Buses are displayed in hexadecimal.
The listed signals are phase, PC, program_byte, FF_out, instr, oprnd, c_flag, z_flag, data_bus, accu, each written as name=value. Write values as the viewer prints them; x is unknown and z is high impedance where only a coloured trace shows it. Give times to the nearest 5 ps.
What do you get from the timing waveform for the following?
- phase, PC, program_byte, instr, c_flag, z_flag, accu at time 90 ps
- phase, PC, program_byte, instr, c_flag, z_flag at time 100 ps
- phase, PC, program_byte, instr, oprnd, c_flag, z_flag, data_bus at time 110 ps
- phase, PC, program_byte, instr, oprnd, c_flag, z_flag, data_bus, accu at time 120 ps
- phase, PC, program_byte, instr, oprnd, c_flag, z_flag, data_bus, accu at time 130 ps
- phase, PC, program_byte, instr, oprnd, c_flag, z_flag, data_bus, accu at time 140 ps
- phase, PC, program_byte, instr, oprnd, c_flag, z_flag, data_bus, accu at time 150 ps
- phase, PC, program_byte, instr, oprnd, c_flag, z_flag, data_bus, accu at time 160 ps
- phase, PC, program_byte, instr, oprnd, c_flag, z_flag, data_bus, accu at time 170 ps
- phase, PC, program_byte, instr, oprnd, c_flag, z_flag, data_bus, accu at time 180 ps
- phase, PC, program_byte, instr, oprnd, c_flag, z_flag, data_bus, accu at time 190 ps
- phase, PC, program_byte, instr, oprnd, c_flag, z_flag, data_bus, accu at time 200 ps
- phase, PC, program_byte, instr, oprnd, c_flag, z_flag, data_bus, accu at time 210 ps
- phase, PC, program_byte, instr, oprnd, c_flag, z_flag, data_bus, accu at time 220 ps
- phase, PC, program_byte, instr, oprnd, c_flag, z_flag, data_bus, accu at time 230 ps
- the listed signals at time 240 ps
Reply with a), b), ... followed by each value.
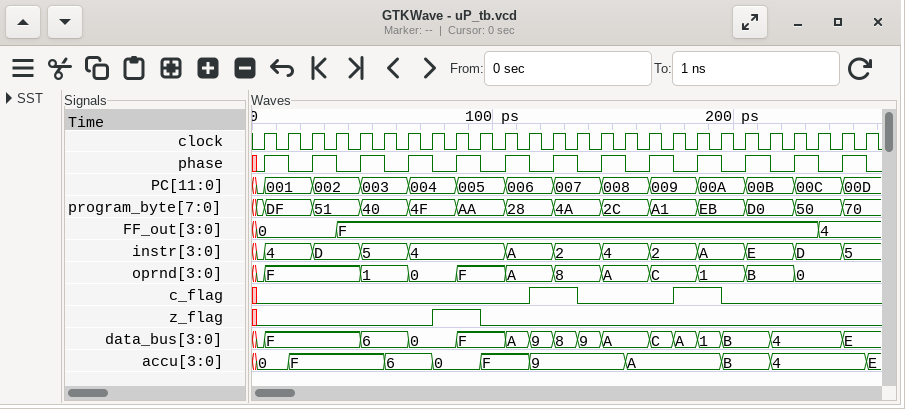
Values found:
a) phase=1, PC=005, program_byte=AA, instr=4, c_flag=0, z_flag=1, accu=0
b) phase=0, PC=005, program_byte=AA, instr=4, c_flag=0, z_flag=0
c) phase=1, PC=006, program_byte=28, instr=A, oprnd=A, c_flag=0, z_flag=0, data_bus=A
d) phase=0, PC=006, program_byte=28, instr=A, oprnd=A, c_flag=1, z_flag=0, data_bus=9, accu=9
e) phase=1, PC=007, program_byte=4A, instr=2, oprnd=8, c_flag=1, z_flag=0, data_bus=8, accu=9
f) phase=0, PC=007, program_byte=4A, instr=2, oprnd=8, c_flag=0, z_flag=0, data_bus=9, accu=9
g) phase=1, PC=008, program_byte=2C, instr=4, oprnd=A, c_flag=0, z_flag=0, data_bus=A, accu=9
h) phase=0, PC=008, program_byte=2C, instr=4, oprnd=A, c_flag=0, z_flag=0, data_bus=A, accu=A
i) phase=1, PC=009, program_byte=A1, instr=2, oprnd=C, c_flag=0, z_flag=0, data_bus=C, accu=A
j) phase=0, PC=009, program_byte=A1, instr=2, oprnd=C, c_flag=1, z_flag=0, data_bus=A, accu=A
k) phase=1, PC=00A, program_byte=EB, instr=A, oprnd=1, c_flag=1, z_flag=0, data_bus=1, accu=A
l) phase=0, PC=00A, program_byte=EB, instr=A, oprnd=1, c_flag=0, z_flag=0, data_bus=B, accu=B
m) phase=1, PC=00B, program_byte=D0, instr=E, oprnd=B, c_flag=0, z_flag=0, data_bus=B, accu=B
n) phase=0, PC=00B, program_byte=D0, instr=E, oprnd=B, c_flag=0, z_flag=0, data_bus=4, accu=4
o) phase=1, PC=00C, program_byte=50, instr=D, oprnd=0, c_flag=0, z_flag=0, data_bus=4, accu=4
p) phase=0, PC=00C, program_byte=50, FF_out=4, instr=D, oprnd=0, c_flag=0, z_flag=0, data_bus=4, accu=4
